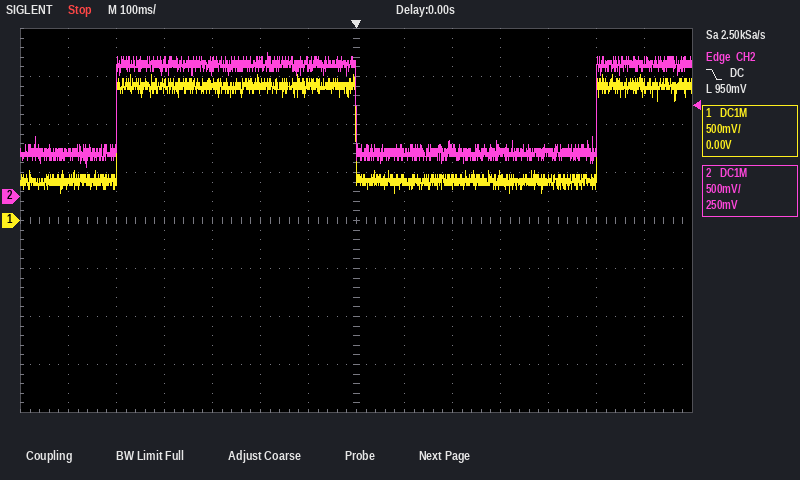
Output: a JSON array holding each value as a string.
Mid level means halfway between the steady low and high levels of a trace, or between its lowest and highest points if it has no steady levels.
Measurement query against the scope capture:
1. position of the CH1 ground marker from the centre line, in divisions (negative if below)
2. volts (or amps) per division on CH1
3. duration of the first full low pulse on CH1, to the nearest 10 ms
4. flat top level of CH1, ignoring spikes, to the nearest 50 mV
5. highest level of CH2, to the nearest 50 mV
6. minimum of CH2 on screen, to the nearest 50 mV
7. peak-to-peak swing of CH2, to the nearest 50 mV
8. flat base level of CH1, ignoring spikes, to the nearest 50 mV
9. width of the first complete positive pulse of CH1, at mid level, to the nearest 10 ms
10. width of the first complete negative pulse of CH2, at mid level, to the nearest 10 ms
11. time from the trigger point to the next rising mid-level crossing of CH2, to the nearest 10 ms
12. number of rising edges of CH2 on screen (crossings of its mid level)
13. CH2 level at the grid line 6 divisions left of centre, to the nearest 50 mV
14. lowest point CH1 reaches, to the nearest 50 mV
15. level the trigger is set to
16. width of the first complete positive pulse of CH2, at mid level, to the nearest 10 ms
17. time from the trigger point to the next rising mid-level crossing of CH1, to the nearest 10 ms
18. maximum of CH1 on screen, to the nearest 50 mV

["0.0 div", "500 mV", "500 ms", "1.40 V", "1.50 V", "300 mV", "1.20 V", "400 mV", "500 ms", "500 ms", "500 ms", "2", "450 mV", "300 mV", "950 mV", "500 ms", "500 ms", "1.50 V"]
